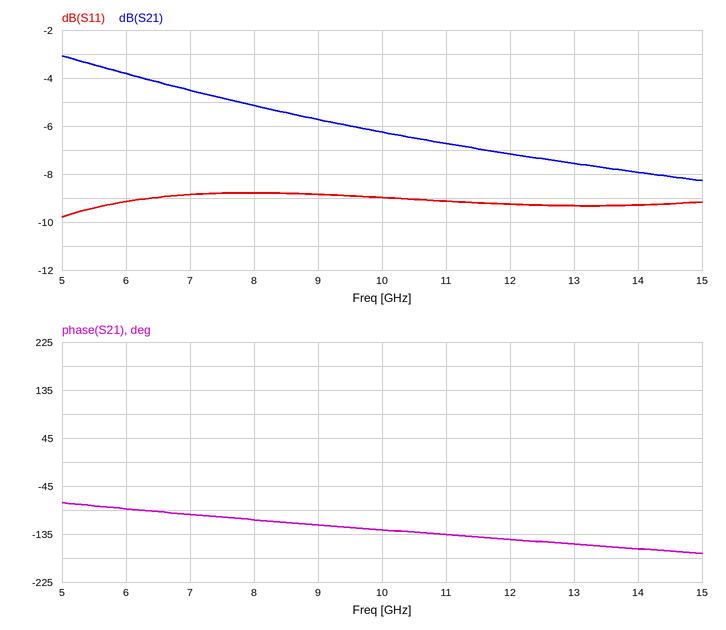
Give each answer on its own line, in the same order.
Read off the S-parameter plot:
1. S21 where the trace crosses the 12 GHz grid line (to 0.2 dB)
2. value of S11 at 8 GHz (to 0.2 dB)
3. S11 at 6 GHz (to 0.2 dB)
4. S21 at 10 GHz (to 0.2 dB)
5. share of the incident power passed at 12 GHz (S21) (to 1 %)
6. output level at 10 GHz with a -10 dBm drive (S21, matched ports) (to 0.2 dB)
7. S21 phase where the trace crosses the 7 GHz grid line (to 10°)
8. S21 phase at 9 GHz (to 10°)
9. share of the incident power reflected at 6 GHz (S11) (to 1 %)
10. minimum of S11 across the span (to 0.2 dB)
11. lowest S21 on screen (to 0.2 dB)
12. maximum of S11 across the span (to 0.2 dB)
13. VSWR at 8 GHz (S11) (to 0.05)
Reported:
-7.2 dB
-8.8 dB
-9.2 dB
-6.2 dB
19 %
-16.2 dBm
-100°
-120°
12 %
-9.8 dB
-8.2 dB
-8.8 dB
2.15
